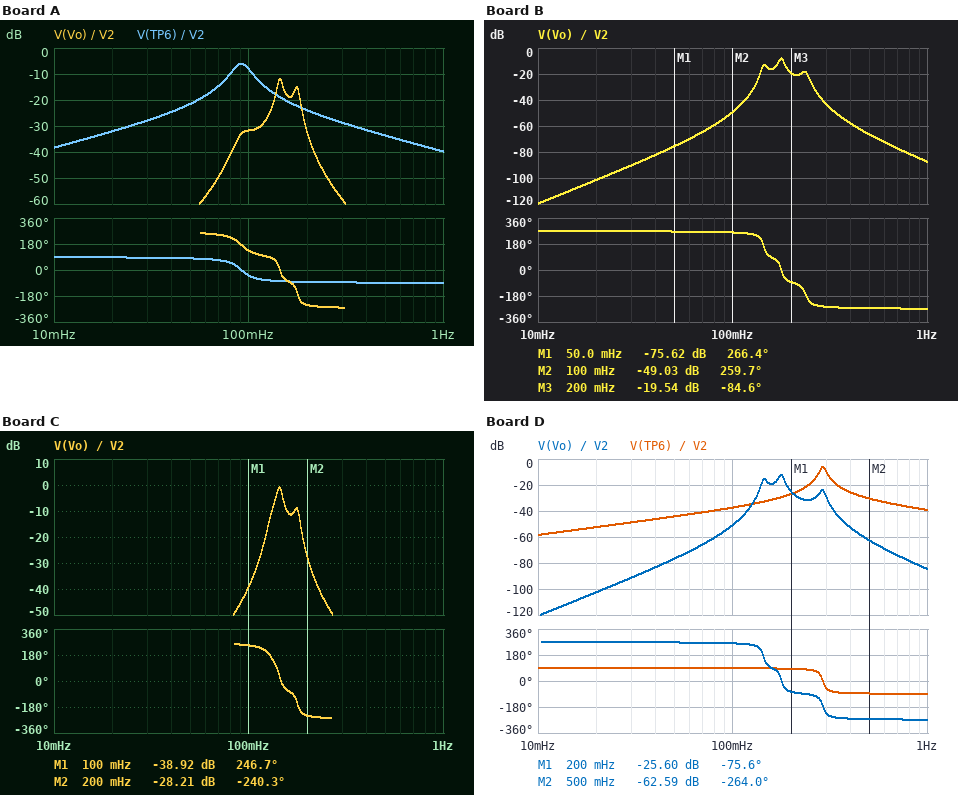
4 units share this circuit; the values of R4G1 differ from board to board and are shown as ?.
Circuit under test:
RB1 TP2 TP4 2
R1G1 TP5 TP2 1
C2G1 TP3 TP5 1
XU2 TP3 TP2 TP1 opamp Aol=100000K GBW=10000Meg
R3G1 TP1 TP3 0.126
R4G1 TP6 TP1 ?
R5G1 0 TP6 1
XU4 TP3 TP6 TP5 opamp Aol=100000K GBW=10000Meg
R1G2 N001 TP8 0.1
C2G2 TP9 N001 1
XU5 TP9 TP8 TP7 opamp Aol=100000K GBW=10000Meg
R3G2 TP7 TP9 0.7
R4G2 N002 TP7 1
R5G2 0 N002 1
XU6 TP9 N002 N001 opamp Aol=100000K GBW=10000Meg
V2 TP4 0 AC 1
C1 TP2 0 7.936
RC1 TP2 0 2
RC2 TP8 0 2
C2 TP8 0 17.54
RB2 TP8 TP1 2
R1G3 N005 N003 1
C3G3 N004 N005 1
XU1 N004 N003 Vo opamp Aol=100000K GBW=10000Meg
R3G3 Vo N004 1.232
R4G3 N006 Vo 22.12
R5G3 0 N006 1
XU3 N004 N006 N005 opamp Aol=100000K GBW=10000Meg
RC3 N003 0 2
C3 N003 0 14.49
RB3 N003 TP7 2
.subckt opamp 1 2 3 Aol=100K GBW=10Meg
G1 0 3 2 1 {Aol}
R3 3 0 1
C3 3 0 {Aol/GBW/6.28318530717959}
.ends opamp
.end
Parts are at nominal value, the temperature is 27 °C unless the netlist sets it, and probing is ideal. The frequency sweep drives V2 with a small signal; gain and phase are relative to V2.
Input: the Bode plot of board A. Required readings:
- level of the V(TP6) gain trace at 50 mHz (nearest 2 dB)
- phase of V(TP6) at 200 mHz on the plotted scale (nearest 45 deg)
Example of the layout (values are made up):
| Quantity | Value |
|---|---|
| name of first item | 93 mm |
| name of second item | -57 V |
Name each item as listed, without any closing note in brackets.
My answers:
| Quantity | Value |
|---|---|
| level of the V(TP6) gain trace at 50 mHz | -22 dB |
| phase of V(TP6) at 200 mHz on the plotted scale | -90 deg |
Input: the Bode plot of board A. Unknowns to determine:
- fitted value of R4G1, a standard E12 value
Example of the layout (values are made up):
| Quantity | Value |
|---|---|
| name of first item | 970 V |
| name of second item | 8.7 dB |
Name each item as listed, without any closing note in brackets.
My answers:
| Quantity | Value |
|---|---|
| fitted value of R4G1, a standard E12 value | 0.33 Ω |
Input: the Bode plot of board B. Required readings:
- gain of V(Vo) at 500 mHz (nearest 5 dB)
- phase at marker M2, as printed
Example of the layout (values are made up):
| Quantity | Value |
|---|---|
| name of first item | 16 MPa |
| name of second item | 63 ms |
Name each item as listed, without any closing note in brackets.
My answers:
| Quantity | Value |
|---|---|
| gain of V(Vo) at 500 mHz | -65 dB |
| phase at marker M2, as printed | 259.7 deg |
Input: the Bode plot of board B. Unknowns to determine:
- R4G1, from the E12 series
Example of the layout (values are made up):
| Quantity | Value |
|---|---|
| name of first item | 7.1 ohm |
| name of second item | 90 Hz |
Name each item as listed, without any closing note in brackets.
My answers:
| Quantity | Value |
|---|---|
| R4G1, from the E12 series | 2.2 Ω |
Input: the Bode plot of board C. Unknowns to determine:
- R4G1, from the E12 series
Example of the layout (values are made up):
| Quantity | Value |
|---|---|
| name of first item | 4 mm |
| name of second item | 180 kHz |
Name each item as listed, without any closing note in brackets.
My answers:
| Quantity | Value |
|---|---|
| R4G1, from the E12 series | 0.68 Ω |
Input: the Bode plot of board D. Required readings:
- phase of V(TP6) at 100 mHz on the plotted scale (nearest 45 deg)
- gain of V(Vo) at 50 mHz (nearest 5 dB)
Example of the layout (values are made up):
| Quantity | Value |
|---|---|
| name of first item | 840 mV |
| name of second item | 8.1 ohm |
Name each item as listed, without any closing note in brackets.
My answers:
| Quantity | Value |
|---|---|
| phase of V(TP6) at 100 mHz on the plotted scale | 90 deg |
| gain of V(Vo) at 50 mHz | -75 dB |
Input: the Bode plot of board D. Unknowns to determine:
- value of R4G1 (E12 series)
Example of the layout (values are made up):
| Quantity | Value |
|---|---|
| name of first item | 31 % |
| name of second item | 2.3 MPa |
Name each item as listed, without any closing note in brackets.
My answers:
| Quantity | Value |
|---|---|
| value of R4G1 | 3.3 Ω |
